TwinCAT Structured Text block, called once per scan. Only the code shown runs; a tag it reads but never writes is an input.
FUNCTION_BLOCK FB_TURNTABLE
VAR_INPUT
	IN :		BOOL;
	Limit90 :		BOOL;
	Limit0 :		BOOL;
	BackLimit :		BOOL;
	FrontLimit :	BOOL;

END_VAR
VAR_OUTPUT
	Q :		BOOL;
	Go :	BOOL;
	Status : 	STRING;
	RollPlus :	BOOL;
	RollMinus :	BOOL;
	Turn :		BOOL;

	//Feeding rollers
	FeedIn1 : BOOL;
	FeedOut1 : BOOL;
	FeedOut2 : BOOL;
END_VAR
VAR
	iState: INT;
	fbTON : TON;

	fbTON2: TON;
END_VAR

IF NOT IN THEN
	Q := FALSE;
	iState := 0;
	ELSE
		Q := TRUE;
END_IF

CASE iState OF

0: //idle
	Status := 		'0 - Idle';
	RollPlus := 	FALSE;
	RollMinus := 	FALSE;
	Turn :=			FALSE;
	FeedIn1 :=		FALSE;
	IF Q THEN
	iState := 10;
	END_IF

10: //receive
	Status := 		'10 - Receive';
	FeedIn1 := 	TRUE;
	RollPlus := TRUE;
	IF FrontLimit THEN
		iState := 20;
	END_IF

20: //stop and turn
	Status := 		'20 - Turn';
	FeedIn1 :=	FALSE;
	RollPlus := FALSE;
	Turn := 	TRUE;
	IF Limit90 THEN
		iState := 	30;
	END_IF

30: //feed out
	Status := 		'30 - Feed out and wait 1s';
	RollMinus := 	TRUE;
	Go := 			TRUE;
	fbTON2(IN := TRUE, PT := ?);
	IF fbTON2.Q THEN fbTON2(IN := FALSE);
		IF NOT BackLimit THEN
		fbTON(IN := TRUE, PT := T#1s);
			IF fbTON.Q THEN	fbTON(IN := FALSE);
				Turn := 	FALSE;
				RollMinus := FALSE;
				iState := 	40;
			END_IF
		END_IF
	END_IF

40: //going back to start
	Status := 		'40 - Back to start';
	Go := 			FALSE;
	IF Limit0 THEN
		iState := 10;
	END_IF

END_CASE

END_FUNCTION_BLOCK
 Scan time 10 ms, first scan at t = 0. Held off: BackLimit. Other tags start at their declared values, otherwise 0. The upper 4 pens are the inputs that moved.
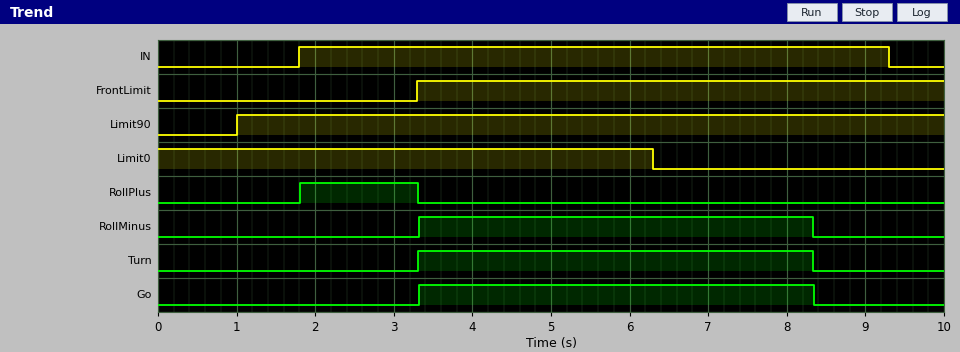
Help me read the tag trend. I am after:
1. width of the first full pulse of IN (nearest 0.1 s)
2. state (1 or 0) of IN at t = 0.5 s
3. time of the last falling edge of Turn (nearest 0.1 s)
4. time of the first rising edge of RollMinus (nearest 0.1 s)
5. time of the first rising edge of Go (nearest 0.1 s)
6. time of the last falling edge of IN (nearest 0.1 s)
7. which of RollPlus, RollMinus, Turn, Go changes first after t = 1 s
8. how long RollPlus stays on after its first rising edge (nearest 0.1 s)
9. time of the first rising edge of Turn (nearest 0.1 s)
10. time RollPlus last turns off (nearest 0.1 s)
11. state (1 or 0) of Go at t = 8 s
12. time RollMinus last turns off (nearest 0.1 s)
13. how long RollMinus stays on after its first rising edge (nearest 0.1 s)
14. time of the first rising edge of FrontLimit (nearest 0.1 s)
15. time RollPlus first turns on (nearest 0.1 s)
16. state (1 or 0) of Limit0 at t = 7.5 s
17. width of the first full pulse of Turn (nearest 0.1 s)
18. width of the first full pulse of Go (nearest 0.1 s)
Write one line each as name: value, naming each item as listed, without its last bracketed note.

width of the first full pulse of IN: 7.5 s
state (1 or 0) of IN at t = 0.5 s: 0
time of the last falling edge of Turn: 8.3 s
time of the first rising edge of RollMinus: 3.3 s
time of the first rising edge of Go: 3.3 s
time of the last falling edge of IN: 9.3 s
which of RollPlus, RollMinus, Turn, Go changes first after t = 1 s: RollPlus
how long RollPlus stays on after its first rising edge: 1.5 s
time of the first rising edge of Turn: 3.3 s
time RollPlus last turns off: 3.3 s
state (1 or 0) of Go at t = 8 s: 1
time RollMinus last turns off: 8.3 s
how long RollMinus stays on after its first rising edge: 5.0 s
time of the first rising edge of FrontLimit: 3.3 s
time RollPlus first turns on: 1.8 s
state (1 or 0) of Limit0 at t = 7.5 s: 0
width of the first full pulse of Turn: 5.0 s
width of the first full pulse of Go: 5.0 s
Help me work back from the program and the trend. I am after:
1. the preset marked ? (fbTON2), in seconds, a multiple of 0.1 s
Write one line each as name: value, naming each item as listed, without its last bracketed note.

the preset marked ? (fbTON2), in seconds, a multiple of 0.1 s: 2.5 s
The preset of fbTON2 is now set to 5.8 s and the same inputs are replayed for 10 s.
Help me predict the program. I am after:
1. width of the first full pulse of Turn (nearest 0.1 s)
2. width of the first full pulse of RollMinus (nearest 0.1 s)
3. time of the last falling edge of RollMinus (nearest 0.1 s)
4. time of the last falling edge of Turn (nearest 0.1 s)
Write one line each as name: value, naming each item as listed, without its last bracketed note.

width of the first full pulse of Turn: 6.0 s
width of the first full pulse of RollMinus: 6.0 s
time of the last falling edge of RollMinus: 9.3 s
time of the last falling edge of Turn: 9.3 s
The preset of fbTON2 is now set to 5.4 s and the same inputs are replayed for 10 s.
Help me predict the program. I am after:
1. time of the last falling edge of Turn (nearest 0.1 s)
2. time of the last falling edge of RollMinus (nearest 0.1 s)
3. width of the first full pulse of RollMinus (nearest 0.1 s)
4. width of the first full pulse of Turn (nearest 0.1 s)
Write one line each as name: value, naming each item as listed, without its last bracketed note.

time of the last falling edge of Turn: 9.3 s
time of the last falling edge of RollMinus: 9.3 s
width of the first full pulse of RollMinus: 6.0 s
width of the first full pulse of Turn: 6.0 s
